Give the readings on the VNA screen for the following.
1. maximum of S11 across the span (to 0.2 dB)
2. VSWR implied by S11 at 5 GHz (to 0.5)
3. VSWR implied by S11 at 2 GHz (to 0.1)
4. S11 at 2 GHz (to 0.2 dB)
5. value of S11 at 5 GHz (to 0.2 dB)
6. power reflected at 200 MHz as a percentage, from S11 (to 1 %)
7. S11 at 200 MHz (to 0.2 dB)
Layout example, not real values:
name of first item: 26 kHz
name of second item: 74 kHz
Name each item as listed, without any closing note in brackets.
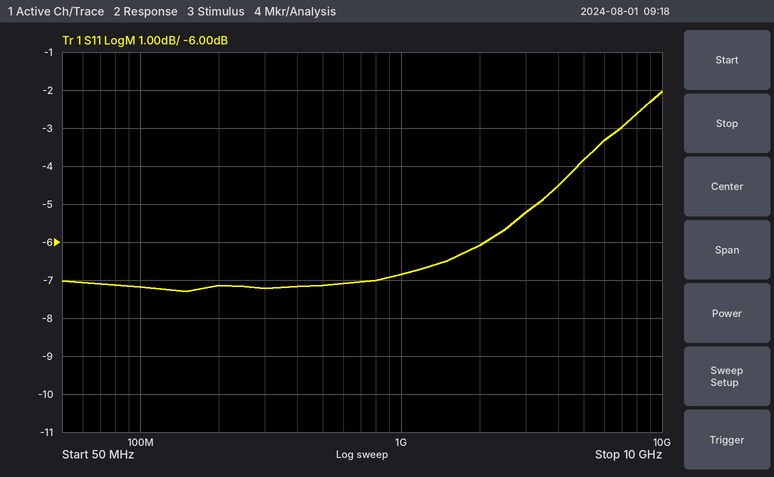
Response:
maximum of S11 across the span: -2.0 dB
VSWR implied by S11 at 5 GHz: 4.5
VSWR implied by S11 at 2 GHz: 3.0
S11 at 2 GHz: -6.0 dB
value of S11 at 5 GHz: -3.8 dB
power reflected at 200 MHz as a percentage, from S11: 19 %
S11 at 200 MHz: -7.2 dB
